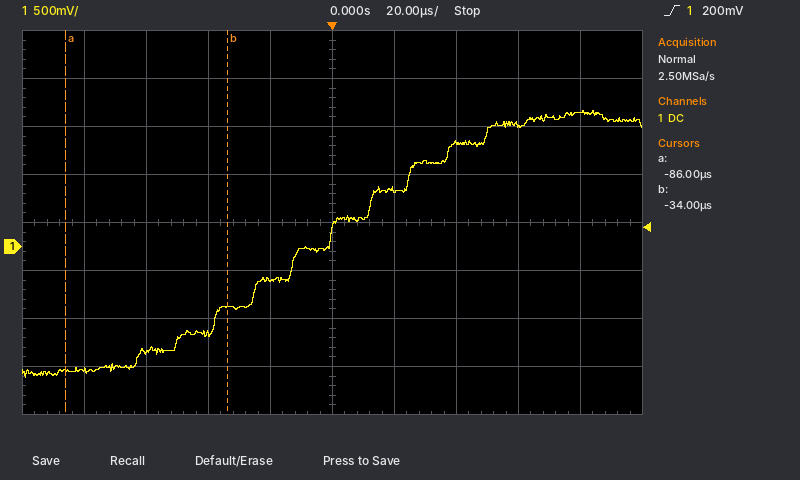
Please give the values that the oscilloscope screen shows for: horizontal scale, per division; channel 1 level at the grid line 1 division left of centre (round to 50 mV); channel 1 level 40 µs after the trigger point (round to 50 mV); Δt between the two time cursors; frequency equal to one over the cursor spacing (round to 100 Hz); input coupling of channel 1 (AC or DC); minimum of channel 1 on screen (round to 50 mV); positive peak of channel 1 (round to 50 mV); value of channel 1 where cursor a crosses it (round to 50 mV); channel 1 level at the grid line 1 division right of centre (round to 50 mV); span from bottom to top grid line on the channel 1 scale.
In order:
20 µs
-350 mV
1.10 V
52 µs
19.2 kHz
DC
-1.35 V
1.40 V
-1.30 V
600 mV
4 V
